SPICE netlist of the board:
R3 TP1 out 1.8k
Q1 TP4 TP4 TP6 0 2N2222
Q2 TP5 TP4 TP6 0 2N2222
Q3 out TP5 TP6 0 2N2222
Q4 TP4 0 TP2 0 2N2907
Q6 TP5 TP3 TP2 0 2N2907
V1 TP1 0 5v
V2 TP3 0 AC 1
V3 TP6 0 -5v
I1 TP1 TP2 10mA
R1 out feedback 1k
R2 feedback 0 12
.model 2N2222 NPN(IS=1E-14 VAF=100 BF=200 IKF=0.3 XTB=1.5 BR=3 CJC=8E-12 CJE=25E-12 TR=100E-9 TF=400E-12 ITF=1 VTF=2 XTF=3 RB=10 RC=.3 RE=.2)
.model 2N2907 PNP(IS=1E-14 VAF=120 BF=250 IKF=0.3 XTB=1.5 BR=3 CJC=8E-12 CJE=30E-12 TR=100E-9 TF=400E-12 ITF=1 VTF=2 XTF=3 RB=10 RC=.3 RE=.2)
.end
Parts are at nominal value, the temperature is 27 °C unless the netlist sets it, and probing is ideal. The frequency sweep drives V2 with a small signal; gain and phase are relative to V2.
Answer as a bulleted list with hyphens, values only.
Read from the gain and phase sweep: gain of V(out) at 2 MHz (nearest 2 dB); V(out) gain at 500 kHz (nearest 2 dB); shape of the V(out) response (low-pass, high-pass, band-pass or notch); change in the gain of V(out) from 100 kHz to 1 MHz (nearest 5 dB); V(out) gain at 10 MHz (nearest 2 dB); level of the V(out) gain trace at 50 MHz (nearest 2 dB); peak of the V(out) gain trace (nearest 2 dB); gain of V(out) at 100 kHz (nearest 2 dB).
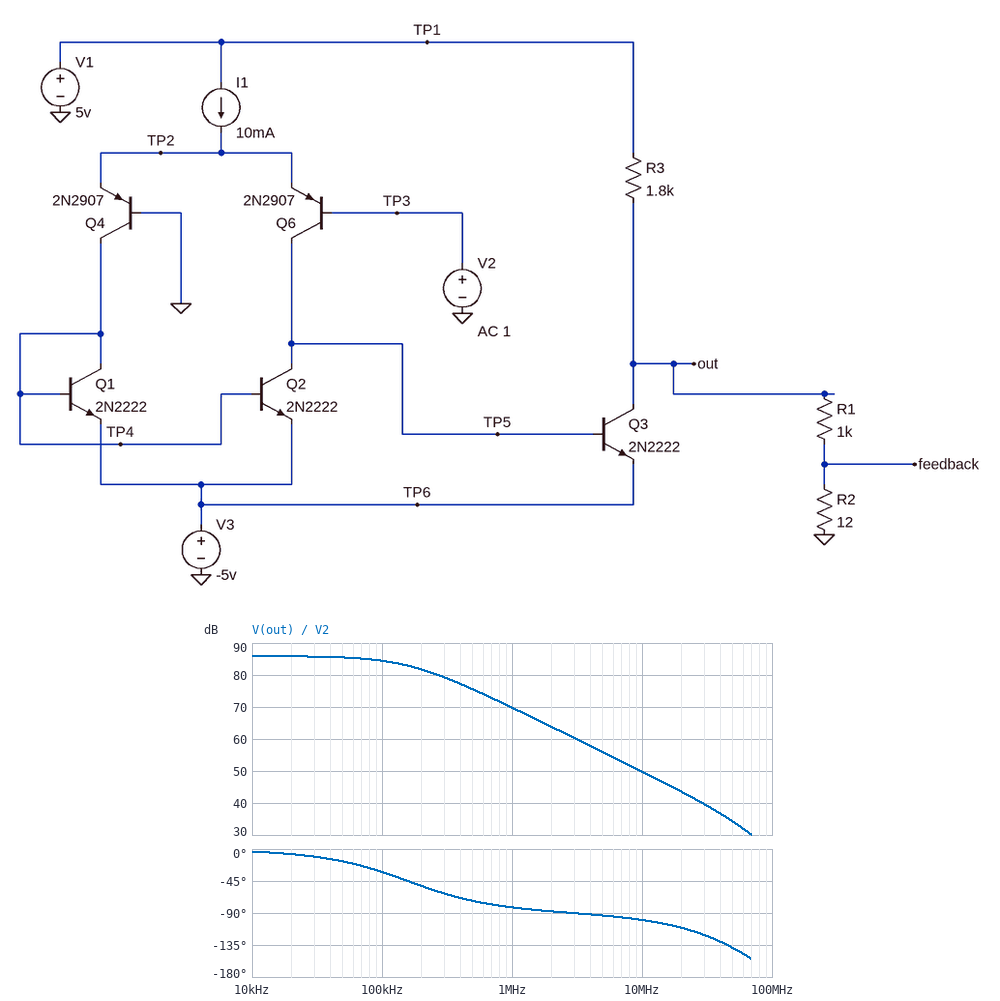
- 64 dB
- 76 dB
- low-pass
- -15 dB
- 50 dB
- 34 dB
- 86 dB
- 84 dB
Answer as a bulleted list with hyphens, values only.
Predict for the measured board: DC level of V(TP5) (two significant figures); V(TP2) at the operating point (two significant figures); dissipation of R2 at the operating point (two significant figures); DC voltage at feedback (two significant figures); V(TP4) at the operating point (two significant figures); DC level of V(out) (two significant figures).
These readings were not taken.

- -4.3 V
- 700 mV
- 220 µW
- -51 mV
- -4.3 V
- -4.3 V
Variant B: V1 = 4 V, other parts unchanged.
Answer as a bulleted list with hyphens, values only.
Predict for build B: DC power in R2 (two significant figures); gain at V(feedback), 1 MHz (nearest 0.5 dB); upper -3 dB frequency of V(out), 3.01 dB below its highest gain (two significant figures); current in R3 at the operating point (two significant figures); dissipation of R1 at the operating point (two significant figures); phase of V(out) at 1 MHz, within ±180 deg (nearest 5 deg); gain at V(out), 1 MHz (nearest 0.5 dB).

- 250 µW
- 29.5 dB
- 130 kHz
- 4.8 mA
- 21 mW
- -85 deg
- 68.0 dB
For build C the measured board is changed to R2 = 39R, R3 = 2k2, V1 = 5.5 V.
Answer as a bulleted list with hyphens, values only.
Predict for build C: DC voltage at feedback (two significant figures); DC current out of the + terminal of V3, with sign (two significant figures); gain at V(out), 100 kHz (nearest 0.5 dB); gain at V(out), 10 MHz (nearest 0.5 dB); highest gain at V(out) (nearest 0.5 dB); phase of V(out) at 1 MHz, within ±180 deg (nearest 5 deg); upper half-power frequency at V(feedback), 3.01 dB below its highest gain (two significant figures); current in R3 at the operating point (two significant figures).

- -180 mV
- -19 mA
- 74.5 dB
- 43.5 dB
- 75.0 dB
- -75 deg
- 260 kHz
- 4.7 mA
